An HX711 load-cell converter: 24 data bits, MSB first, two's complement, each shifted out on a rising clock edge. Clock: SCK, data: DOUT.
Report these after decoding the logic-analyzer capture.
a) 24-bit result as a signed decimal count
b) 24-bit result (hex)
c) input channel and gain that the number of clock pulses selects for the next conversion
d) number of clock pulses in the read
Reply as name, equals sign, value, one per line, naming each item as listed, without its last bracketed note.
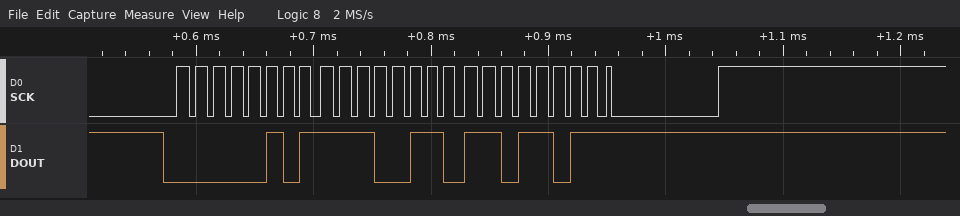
24-bit result as a signed decimal count = 386779
24-bit result = 0x05E6DB
input channel and gain that the number of clock pulses selects for the next conversion = channel B, gain 32
number of clock pulses in the read = 26
